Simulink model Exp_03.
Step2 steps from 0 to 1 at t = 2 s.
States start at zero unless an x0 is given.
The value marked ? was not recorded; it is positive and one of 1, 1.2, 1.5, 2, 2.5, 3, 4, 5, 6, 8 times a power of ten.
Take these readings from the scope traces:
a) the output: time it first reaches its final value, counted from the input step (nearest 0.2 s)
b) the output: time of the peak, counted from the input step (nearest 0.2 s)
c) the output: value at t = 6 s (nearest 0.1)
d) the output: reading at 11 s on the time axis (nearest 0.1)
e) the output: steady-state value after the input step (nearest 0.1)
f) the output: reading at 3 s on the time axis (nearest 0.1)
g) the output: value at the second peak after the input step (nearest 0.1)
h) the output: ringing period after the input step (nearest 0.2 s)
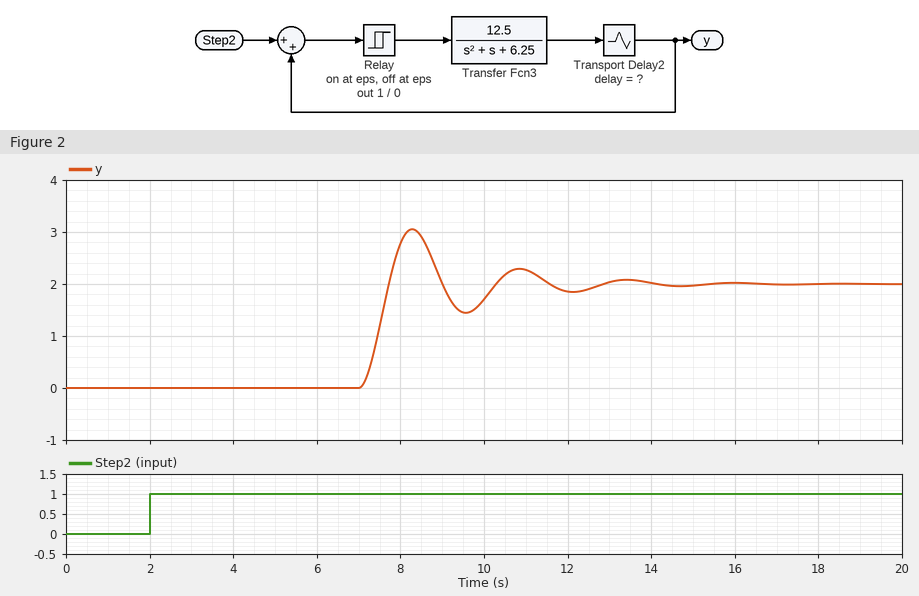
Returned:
5.8 s
6.2 s
0.0
2.3
2.0
0.0
2.3
2.6 s
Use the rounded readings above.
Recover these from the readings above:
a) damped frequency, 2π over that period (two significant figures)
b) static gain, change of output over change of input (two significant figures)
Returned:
2.4 rad/s
2.0
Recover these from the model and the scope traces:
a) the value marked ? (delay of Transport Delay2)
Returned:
5
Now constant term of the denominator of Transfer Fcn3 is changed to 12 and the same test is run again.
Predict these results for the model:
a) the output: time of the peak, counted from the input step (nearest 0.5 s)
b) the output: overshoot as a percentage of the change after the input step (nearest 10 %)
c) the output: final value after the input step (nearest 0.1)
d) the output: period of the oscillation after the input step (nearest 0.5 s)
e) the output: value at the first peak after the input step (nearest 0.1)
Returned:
6.0 s
60 %
1.0
2.0 s
1.7
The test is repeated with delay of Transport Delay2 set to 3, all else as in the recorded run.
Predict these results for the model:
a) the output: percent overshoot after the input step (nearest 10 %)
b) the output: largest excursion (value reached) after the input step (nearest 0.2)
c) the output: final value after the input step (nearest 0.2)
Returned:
50 %
3.0
2.0
